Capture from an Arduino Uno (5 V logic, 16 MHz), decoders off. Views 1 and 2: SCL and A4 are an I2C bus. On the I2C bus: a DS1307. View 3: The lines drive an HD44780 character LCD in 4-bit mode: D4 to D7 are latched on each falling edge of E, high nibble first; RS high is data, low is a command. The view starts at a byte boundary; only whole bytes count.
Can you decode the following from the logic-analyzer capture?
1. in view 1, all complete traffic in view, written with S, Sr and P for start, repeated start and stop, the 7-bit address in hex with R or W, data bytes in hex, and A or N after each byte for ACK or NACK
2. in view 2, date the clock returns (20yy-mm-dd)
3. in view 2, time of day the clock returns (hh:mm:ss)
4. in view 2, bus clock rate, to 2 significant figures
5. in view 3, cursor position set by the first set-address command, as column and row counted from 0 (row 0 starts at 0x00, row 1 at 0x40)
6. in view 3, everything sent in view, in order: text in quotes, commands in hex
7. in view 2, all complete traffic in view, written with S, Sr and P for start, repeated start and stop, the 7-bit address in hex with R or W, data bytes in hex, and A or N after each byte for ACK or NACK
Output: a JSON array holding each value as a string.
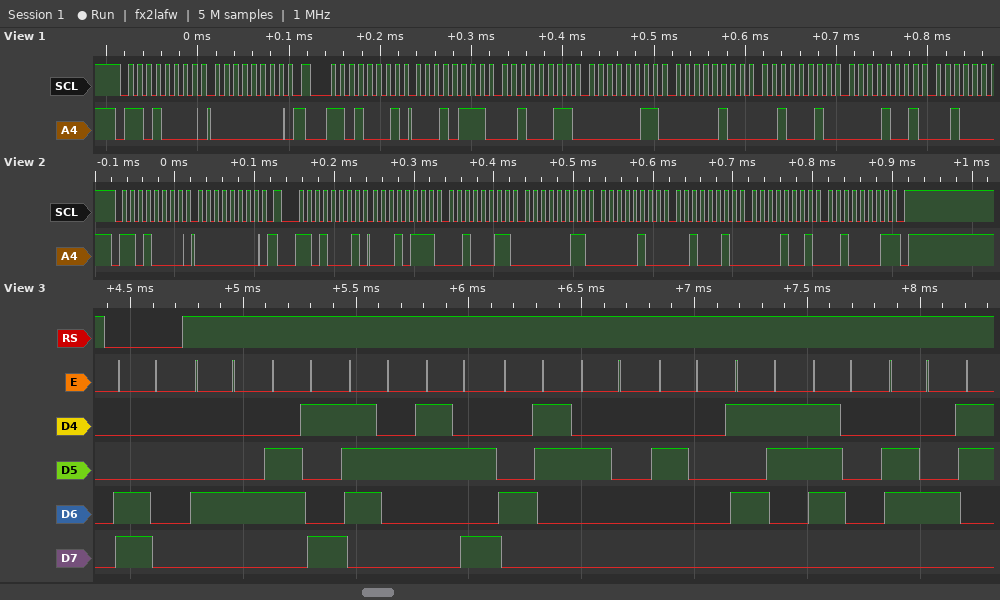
["S 68W A 00 A Sr 68R A 17 A 23 A 03 A 04 A 22 A 09 A", "2021-09-22", "03:23:17", "100 kHz", "column 0, row 1", "0xC0 \"Dir:C  Spd\"", "S 68W A 00 A Sr 68R A 17 A 23 A 03 A 04 A 22 A 09 A 21 N P"]
